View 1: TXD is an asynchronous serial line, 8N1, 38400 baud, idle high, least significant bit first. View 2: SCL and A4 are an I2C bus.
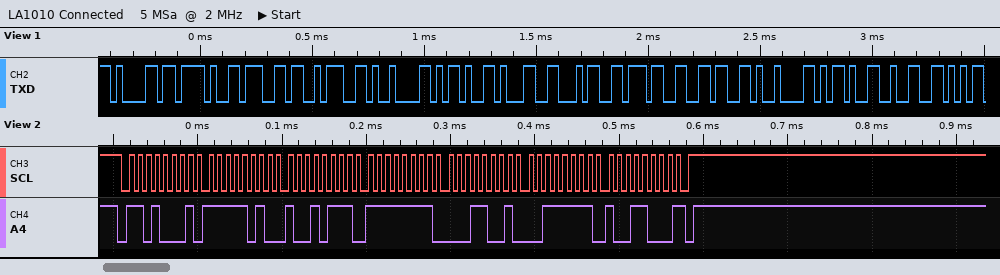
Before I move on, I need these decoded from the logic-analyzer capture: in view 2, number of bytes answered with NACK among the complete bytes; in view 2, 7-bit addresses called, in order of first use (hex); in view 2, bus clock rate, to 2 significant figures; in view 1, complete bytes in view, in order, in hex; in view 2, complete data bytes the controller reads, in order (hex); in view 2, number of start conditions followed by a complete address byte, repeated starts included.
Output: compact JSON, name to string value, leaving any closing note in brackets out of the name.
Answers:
{"in view 2, number of bytes answered with NACK among the complete bytes": "1", "in view 2, 7-bit addresses called, in order of first use": "0x68", "in view 2, bus clock rate, to 2 significant figures": "100 kHz", "in view 1, complete bytes in view, in order, in hex": "61 2F 67 3A 09 2D 31 34 37 36 09 2D 32", "in view 2, complete data bytes the controller reads, in order": "FA 97 FF 19 3F 98", "in view 2, number of start conditions followed by a complete address byte, repeated starts included": "1"}
